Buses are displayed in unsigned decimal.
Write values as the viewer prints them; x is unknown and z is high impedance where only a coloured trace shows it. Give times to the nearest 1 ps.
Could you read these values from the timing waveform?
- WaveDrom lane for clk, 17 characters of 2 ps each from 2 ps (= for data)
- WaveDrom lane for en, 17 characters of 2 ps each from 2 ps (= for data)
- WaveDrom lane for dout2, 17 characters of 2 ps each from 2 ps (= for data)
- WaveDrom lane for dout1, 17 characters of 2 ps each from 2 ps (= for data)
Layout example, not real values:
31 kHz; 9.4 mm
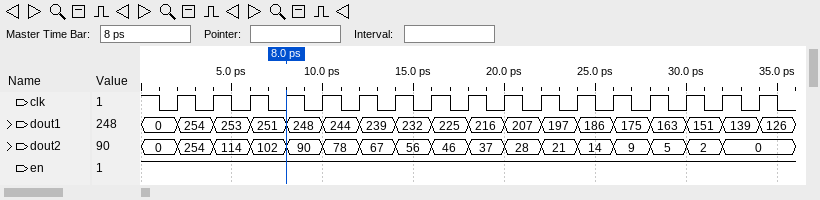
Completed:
{name: 'clk', wave: 'p................'}; {name: 'en', wave: '1................'}; {name: 'dout2', wave: '================.', data: '254 114 102 90 78 67 56 46 37 28 21 14 9 5 2 0'}; {name: 'dout1', wave: '=================', data: '254 253 251 248 244 239 232 225 216 207 197 186 175 163 151 139 126'}
